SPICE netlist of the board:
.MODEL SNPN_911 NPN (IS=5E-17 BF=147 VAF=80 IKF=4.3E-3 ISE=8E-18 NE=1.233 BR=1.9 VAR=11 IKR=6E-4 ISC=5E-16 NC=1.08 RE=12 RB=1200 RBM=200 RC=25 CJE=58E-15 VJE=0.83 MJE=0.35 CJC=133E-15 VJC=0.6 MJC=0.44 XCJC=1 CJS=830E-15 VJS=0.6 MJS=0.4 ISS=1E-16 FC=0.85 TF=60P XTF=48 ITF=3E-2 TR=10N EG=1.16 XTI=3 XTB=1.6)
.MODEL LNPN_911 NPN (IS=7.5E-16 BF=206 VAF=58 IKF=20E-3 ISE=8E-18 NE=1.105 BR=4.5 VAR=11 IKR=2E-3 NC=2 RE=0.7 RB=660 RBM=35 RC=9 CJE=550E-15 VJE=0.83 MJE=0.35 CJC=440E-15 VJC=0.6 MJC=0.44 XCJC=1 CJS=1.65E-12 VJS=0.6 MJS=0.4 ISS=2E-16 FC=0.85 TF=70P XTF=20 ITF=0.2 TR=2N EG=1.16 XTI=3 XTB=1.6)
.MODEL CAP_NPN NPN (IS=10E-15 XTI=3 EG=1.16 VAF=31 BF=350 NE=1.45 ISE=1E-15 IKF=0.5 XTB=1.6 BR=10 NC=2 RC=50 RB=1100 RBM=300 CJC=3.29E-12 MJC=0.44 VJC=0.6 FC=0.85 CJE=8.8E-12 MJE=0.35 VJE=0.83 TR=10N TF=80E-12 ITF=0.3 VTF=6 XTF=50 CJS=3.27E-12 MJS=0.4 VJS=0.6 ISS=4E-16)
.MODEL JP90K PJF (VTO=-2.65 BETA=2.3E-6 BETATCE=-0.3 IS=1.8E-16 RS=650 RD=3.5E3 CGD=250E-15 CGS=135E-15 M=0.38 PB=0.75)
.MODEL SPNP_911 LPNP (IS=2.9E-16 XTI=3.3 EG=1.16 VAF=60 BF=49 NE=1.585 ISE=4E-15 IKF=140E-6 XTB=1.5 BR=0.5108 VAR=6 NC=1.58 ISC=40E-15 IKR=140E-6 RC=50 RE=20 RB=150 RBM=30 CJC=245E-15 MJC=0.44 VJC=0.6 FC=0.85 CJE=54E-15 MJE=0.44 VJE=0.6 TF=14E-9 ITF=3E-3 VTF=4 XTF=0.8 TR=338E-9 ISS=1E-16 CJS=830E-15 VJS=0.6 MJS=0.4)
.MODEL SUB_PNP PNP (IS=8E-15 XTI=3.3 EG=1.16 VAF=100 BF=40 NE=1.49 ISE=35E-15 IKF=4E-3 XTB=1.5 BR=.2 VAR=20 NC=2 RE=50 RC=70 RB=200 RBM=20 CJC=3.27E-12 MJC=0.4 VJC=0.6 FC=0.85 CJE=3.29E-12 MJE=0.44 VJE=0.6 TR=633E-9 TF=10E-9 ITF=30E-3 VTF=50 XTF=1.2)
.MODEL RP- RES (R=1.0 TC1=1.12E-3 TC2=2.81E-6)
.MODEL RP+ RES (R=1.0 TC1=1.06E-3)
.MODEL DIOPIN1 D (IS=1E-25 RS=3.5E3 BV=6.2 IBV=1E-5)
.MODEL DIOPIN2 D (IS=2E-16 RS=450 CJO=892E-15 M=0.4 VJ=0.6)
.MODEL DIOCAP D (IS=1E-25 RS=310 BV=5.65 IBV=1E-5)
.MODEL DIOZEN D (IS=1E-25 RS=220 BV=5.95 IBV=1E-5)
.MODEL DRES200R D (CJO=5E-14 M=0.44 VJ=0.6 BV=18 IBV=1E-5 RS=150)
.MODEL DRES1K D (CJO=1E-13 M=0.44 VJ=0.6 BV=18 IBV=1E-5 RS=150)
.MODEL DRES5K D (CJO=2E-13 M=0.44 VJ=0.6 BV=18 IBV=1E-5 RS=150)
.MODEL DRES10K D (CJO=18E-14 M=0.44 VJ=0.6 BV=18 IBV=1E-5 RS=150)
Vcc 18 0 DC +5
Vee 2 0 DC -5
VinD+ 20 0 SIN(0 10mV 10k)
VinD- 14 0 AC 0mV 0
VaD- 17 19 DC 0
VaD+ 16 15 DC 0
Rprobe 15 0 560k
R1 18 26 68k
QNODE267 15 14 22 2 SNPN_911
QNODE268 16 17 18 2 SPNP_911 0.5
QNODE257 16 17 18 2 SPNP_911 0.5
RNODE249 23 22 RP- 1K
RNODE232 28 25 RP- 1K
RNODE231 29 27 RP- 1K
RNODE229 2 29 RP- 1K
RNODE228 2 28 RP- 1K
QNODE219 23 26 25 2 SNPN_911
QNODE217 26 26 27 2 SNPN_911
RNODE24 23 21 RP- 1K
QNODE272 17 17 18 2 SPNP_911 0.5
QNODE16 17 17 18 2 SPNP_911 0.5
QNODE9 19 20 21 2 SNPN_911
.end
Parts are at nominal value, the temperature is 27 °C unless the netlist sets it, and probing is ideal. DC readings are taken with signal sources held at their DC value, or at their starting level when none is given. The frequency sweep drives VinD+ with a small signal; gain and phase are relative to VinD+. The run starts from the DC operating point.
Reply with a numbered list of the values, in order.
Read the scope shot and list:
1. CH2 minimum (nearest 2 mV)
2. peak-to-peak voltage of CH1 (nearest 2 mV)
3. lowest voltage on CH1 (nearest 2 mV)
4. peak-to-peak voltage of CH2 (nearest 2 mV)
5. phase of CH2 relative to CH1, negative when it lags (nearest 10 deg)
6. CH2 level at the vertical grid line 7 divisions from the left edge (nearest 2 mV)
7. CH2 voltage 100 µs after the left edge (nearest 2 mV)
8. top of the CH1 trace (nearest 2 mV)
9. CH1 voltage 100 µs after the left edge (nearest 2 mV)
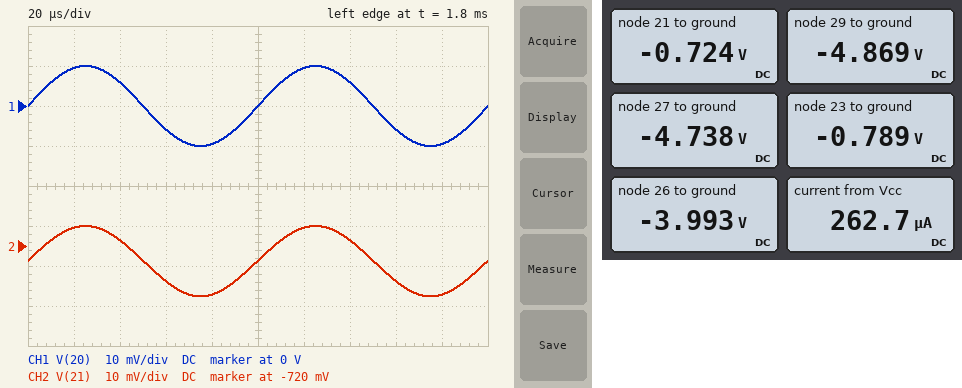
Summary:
1. -732 mV
2. 20 mV
3. -10 mV
4. 18 mV
5. 0 deg
6. -718 mV
7. -724 mV
8. 10 mV
9. 0 V
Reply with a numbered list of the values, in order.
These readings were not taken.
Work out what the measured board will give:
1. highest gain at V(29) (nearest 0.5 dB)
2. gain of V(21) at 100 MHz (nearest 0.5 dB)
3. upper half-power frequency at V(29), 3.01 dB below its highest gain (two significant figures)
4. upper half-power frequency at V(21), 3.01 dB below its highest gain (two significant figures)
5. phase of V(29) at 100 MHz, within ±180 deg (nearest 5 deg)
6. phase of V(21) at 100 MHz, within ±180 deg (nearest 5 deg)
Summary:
1. -35.5 dB
2. -1.5 dB
3. 510 MHz
4. 810 MHz
5. 30 deg
6. -5 deg
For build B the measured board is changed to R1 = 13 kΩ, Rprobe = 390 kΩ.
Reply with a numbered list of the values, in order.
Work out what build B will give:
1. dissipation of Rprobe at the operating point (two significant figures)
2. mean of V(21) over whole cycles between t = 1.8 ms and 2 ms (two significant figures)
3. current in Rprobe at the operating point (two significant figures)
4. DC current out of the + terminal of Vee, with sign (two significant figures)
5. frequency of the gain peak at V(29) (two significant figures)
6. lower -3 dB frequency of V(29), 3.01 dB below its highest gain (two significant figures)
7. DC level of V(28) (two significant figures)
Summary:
1. 1.1 µW
2. -770 mV
3. 1.7 µA
4. -1.2 mA
5. 230 MHz
6. 90 MHz
7. -4.4 V
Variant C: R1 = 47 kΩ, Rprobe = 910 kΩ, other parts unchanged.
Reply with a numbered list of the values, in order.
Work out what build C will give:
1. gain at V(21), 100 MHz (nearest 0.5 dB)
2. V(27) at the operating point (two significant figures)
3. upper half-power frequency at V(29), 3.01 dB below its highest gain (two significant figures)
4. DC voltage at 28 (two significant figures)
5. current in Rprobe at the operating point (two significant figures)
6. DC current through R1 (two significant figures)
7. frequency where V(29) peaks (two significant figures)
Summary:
1. -1.0 dB
2. -4.6 V
3. 540 MHz
4. -4.8 V
5. 320 nA
6. 190 µA
7. 220 MHz
